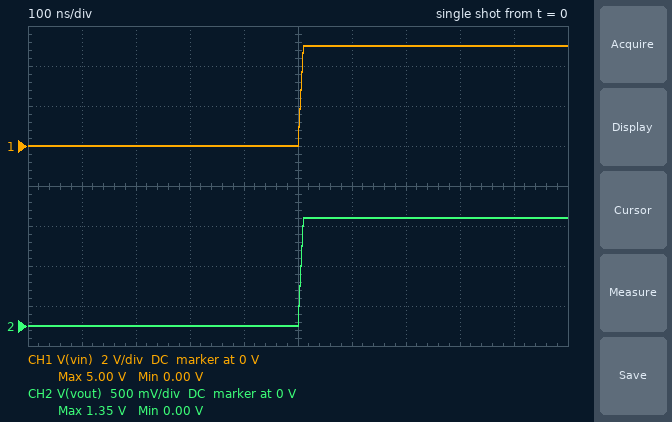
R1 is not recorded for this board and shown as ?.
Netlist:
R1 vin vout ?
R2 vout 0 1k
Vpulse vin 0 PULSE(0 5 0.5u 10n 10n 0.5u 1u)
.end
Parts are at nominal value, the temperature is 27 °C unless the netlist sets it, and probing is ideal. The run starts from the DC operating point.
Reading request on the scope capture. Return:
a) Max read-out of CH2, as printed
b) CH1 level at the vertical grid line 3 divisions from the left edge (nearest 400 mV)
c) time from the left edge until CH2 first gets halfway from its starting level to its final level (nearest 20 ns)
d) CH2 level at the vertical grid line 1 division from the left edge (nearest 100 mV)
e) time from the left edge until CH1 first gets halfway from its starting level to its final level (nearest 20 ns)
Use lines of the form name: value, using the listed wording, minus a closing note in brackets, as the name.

Max read-out of CH2, as printed: 1.35 V
CH1 level at the vertical grid line 3 divisions from the left edge: 0 V
time from the left edge until CH2 first gets halfway from its starting level to its final level: 500 ns
CH2 level at the vertical grid line 1 division from the left edge: 0 V
time from the left edge until CH1 first gets halfway from its starting level to its final level: 500 ns
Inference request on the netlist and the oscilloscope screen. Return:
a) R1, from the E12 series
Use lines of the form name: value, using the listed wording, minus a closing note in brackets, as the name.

R1, from the E12 series: 2.7 kΩ
